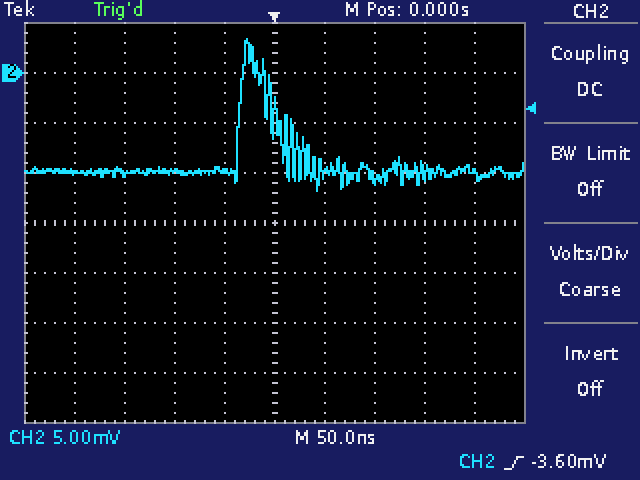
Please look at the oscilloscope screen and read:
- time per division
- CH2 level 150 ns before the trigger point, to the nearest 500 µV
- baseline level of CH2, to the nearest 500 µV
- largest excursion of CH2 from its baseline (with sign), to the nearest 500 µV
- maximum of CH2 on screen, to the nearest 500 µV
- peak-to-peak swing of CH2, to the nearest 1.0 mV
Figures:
50 ns
-10.0 mV
-10.0 mV
+13.5 mV
3.5 mV
15.0 mV
